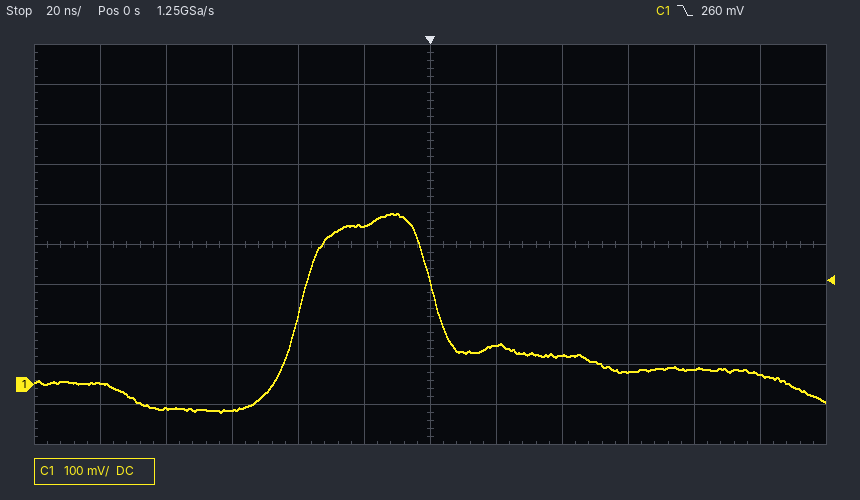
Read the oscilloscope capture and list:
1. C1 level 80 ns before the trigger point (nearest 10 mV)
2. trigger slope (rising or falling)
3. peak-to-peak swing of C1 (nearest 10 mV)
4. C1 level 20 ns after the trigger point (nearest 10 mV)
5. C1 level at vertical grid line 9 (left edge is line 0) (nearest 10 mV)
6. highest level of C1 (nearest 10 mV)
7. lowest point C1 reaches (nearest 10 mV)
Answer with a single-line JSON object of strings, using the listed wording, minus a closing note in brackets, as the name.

{"C1 level 80 ns before the trigger point": "-60 mV", "trigger slope": "falling", "peak-to-peak swing of C1": "500 mV", "C1 level 20 ns after the trigger point": "100 mV", "C1 level at vertical grid line 9 (left edge is line 0)": "30 mV", "highest level of C1": "430 mV", "lowest point C1 reaches": "-70 mV"}
